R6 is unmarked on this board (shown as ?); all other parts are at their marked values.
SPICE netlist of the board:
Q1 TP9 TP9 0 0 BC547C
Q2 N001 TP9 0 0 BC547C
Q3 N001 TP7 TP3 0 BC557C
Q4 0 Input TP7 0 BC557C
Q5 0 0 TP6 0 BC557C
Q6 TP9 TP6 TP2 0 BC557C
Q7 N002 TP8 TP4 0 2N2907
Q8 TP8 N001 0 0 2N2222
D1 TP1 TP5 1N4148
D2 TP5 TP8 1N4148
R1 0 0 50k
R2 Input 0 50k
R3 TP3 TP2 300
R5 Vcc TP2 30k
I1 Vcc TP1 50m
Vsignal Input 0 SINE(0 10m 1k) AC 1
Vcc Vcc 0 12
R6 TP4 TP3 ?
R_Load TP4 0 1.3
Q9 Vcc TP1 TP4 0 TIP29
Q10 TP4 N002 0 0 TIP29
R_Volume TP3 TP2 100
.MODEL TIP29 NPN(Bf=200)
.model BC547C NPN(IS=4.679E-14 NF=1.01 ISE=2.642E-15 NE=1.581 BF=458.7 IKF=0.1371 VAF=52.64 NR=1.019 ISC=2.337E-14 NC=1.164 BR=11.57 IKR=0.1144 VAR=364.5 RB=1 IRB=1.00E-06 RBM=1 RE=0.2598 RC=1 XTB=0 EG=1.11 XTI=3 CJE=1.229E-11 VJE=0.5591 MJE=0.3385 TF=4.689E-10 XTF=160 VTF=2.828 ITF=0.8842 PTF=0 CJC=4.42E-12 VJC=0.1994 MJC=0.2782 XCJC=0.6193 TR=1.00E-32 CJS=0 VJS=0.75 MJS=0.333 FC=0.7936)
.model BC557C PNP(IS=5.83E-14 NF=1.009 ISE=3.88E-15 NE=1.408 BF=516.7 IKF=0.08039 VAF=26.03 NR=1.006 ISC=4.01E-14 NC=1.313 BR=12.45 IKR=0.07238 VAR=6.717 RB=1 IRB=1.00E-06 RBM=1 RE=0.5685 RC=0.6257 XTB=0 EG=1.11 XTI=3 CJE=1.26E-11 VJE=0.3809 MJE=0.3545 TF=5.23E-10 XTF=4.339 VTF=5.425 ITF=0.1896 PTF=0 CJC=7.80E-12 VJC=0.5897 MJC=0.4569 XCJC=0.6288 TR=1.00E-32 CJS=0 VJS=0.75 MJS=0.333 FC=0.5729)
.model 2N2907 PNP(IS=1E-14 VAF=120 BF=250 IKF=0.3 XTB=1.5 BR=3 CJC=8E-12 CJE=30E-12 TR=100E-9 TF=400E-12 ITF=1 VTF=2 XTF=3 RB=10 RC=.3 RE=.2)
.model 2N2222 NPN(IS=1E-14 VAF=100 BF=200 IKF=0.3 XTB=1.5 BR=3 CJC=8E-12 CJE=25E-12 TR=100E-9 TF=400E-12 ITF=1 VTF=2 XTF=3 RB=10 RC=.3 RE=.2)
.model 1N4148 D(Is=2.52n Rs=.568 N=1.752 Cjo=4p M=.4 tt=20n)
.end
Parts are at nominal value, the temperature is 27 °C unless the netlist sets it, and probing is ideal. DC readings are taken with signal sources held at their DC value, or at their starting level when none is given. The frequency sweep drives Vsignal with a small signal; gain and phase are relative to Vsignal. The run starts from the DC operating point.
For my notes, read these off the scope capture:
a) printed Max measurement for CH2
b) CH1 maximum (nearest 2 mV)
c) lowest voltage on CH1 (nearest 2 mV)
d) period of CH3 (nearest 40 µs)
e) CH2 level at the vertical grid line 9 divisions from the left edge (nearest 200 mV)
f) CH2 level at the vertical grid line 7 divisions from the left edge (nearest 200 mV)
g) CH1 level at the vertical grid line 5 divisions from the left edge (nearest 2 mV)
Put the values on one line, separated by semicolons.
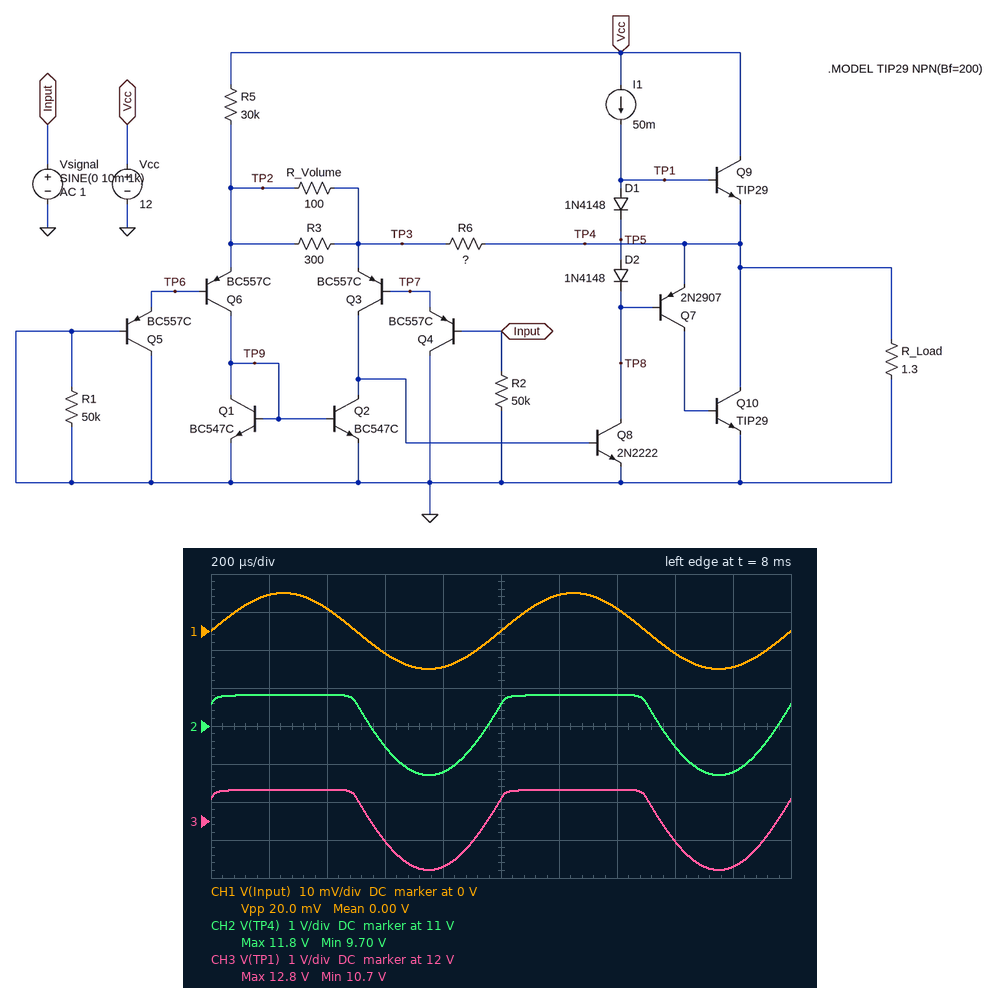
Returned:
11.8 V; 10 mV; -10 mV; 1.00 ms; 9.8 V; 11.8 V; 0 V
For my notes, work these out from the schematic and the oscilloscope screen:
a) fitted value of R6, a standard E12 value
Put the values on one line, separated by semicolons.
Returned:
22 kΩ
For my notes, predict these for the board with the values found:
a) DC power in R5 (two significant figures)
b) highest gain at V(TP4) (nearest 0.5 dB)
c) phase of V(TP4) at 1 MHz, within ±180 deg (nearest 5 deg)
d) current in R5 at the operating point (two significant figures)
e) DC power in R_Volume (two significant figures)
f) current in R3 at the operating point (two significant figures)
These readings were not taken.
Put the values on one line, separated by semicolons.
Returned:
4.0 mW; 46.0 dB; -40 deg; 370 µA; 110 nW; 11 µA
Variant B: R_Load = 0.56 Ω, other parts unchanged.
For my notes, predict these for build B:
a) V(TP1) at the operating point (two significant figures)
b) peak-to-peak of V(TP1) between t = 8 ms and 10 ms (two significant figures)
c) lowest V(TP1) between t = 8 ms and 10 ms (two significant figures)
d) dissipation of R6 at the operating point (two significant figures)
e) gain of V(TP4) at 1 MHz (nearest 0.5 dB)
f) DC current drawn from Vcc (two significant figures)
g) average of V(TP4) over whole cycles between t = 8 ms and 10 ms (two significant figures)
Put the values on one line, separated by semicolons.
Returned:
6.6 V; 360 mV; 6.3 V; 970 µW; -68.0 dB; 10 A; 5.6 V
